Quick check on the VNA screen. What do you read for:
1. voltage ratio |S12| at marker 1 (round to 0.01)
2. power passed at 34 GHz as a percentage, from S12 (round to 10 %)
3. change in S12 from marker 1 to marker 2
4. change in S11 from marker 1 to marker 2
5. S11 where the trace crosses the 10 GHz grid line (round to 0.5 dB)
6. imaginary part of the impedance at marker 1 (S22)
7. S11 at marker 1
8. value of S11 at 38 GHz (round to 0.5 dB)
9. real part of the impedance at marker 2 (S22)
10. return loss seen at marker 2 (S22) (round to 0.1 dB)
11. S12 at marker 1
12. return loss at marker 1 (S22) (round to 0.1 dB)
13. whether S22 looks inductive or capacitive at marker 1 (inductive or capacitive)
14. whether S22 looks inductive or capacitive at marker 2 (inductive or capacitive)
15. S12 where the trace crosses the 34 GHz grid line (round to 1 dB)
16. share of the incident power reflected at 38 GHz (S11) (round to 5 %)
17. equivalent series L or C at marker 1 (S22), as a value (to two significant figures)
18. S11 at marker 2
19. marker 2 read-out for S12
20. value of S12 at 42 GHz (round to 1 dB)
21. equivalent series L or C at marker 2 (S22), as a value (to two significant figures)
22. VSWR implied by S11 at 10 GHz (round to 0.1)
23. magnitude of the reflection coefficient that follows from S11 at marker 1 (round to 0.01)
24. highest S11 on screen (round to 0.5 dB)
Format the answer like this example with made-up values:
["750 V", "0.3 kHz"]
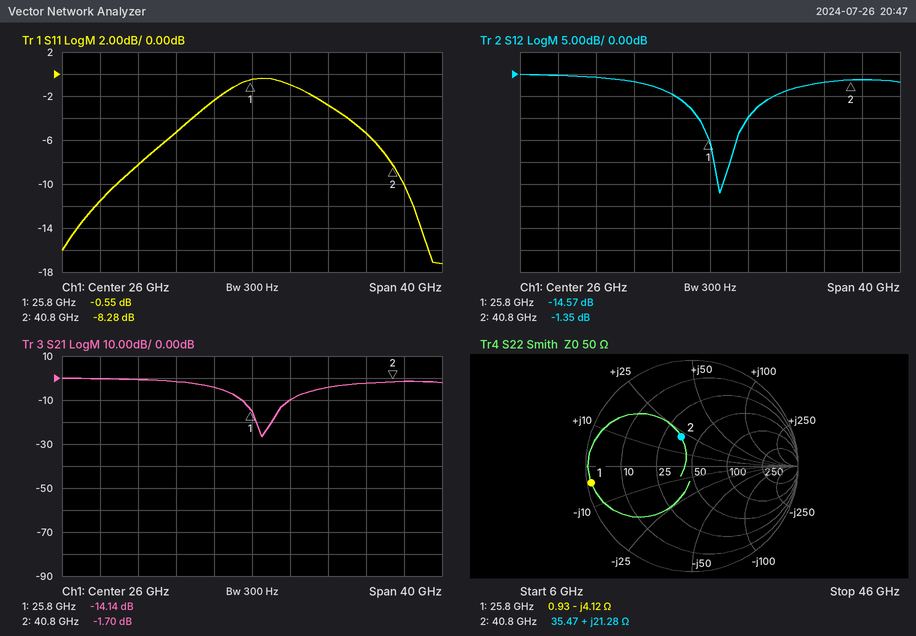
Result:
["0.19", "40 %", "13.22 dB", "-7.73 dB", "-11.5 dB", "-4.12 Ω", "-0.55 dB", "-5.5 dB", "35.47 Ω", "10.7 dB", "-14.57 dB", "0.3 dB", "capacitive", "inductive", "-4 dB", "30 %", "1.5 pF", "-8.28 dB", "-1.35 dB", "-1 dB", "83 pH", "1.7", "0.94", "-0.5 dB"]
